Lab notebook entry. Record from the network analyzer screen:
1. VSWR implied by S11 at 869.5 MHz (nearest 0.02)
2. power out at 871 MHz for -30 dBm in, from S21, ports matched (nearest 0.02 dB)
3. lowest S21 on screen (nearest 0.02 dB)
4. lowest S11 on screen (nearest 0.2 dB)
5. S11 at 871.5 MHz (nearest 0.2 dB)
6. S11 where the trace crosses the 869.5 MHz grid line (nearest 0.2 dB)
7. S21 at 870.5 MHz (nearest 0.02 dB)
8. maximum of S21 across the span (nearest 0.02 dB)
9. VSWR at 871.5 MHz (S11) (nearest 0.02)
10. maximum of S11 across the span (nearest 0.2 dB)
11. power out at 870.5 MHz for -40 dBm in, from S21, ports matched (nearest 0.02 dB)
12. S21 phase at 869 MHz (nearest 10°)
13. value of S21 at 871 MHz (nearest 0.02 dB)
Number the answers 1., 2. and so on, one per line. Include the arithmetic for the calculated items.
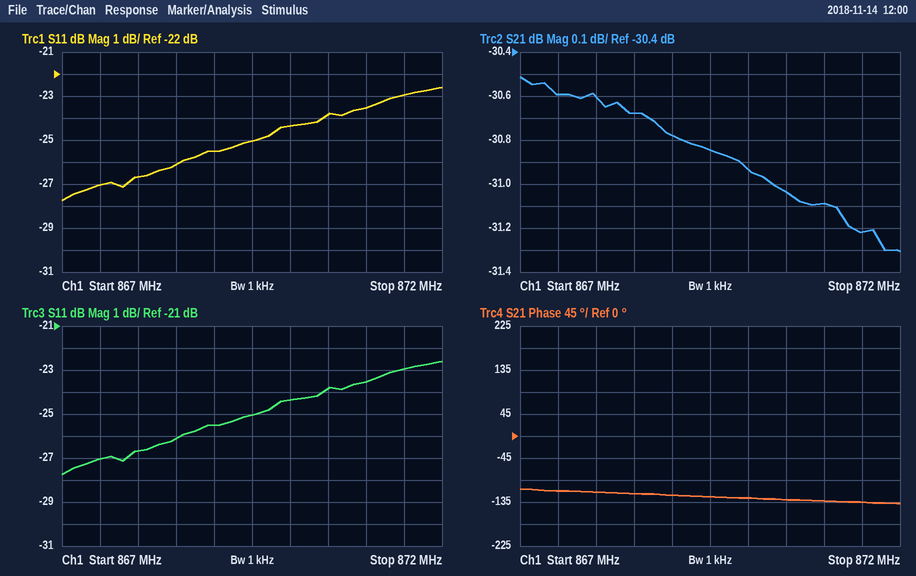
1. |Γ| = 10^(-25/20) = 0.0562; VSWR = (1 + 0.0562)/(1 − 0.0562) ≈ 1.12
2. -30 dBm + (-31.08 dB) = -61.08 dBm
3. -31.30 dB
4. -27.8 dB
5. -23.0 dB
6. -25.0 dB
7. -31.04 dB
8. -30.52 dB
9. |Γ| = 10^(-23/20) = 0.0708; VSWR = (1 + 0.0708)/(1 − 0.0708) ≈ 1.15, so 1.16 to the nearest 0.02
10. -22.6 dB
11. -40 dBm + (-31.04 dB) = -71.04 dBm
12. -120°
13. -31.08 dB
